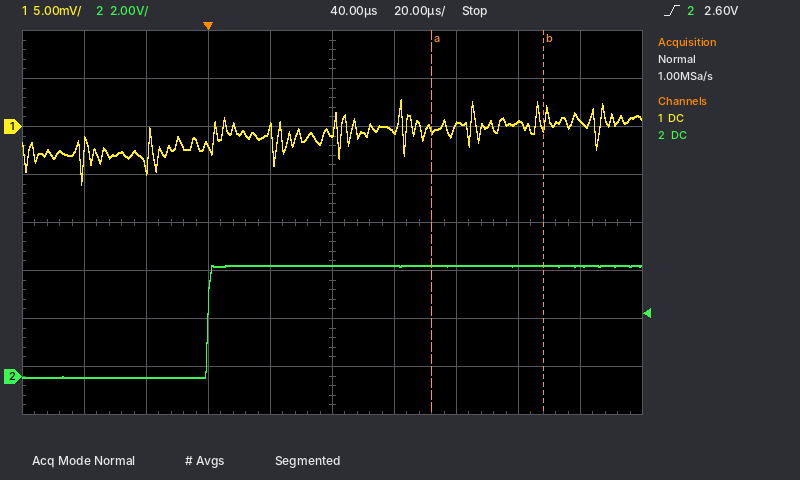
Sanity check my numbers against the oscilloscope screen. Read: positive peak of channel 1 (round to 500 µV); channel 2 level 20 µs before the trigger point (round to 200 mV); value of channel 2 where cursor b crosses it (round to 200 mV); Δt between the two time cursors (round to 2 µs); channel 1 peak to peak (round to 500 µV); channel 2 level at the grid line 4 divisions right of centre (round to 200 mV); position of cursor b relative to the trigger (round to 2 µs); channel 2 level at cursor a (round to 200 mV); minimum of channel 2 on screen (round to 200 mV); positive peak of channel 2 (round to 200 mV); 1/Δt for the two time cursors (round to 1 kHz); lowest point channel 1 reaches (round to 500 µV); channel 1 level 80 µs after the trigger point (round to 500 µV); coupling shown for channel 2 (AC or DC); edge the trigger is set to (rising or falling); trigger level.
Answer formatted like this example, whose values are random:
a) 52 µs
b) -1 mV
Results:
a) 3.0 mV
b) 0.0 V
c) 4.6 V
d) 36 µs
e) 9.0 mV
f) 4.6 V
g) +108 µs
h) 4.6 V
i) 0.0 V
j) 4.6 V
k) 28 kHz
l) -6.0 mV
m) 0.0 mV
n) DC
o) rising
p) 2.60 V
